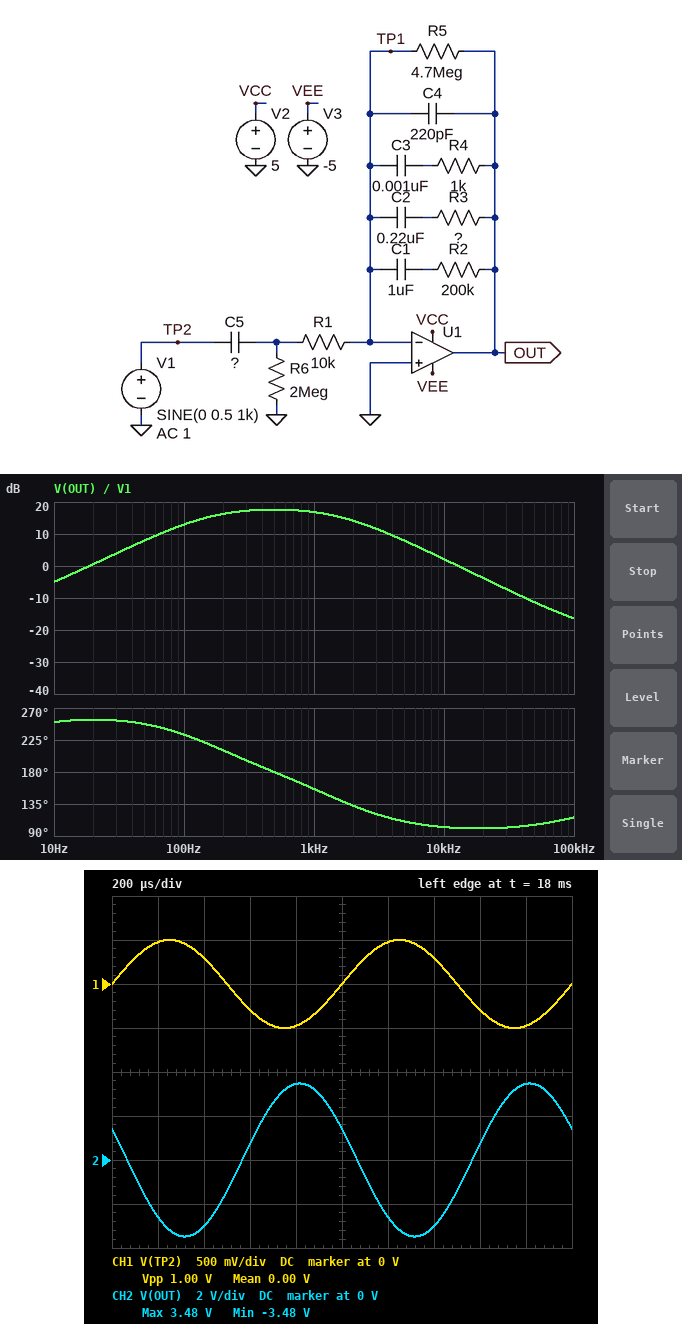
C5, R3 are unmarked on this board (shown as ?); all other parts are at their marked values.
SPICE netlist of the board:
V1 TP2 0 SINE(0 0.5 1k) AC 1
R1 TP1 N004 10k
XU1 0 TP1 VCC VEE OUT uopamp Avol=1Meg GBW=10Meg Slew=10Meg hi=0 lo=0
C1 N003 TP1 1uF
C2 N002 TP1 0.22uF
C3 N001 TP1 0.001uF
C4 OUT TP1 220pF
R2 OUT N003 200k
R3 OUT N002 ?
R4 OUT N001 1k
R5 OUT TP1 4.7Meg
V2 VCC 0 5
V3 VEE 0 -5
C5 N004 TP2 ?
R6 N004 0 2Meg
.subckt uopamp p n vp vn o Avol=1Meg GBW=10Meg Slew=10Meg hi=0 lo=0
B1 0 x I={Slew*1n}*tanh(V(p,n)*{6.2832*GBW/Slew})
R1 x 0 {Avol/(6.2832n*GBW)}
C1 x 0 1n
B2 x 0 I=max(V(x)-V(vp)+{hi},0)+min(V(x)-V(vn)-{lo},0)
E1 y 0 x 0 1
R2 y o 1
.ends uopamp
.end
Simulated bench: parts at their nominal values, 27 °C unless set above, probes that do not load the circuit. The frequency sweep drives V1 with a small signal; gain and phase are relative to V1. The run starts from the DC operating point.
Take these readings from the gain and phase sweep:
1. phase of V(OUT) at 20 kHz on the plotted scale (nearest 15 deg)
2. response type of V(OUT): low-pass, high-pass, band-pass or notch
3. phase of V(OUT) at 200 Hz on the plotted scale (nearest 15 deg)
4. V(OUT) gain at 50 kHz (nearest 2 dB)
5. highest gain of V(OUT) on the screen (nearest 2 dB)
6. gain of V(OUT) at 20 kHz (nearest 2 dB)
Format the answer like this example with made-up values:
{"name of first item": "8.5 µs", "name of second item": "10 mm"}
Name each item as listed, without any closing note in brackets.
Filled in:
{"phase of V(OUT) at 20 kHz on the plotted scale": "105 deg", "response type of V(OUT): low-pass, high-pass, band-pass or notch": "band-pass", "phase of V(OUT) at 200 Hz on the plotted scale": "210 deg", "V(OUT) gain at 50 kHz": "-12 dB", "highest gain of V(OUT) on the screen": "18 dB", "gain of V(OUT) at 20 kHz": "-4 dB"}
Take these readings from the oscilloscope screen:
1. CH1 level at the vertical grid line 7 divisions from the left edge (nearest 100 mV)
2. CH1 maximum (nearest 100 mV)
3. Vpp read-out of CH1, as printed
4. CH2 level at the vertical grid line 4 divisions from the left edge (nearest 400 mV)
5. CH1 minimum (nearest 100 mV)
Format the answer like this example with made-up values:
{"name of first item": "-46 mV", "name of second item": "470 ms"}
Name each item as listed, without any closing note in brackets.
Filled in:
{"CH1 level at the vertical grid line 7 divisions from the left edge": "300 mV", "CH1 maximum": "500 mV", "Vpp read-out of CH1, as printed": "1.00 V", "CH2 level at the vertical grid line 4 divisions from the left edge": "3.6 V", "CH1 minimum": "-500 mV"}
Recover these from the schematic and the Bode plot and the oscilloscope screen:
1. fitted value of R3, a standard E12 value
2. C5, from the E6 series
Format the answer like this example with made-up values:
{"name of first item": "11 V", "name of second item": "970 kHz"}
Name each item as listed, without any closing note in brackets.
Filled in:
{"fitted value of R3, a standard E12 value": "150 kΩ", "C5, from the E6 series": "100 nF"}
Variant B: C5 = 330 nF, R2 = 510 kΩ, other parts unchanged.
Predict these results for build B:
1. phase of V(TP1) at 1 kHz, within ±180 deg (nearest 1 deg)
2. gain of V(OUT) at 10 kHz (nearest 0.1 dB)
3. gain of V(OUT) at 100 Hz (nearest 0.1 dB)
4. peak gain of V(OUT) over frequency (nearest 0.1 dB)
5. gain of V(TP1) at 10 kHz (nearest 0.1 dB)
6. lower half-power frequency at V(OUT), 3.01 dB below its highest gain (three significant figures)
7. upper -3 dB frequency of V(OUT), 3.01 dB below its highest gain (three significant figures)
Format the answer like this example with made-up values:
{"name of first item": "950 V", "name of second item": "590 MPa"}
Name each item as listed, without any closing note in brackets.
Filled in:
{"phase of V(TP1) at 1 kHz, within ±180 deg": "51 deg", "gain of V(OUT) at 10 kHz": "2.2 dB", "gain of V(OUT) at 100 Hz": "20.1 dB", "peak gain of V(OUT) over frequency": "20.7 dB", "gain of V(TP1) at 10 kHz": "-57.8 dB", "lower half-power frequency at V(OUT), 3.01 dB below its highest gain": "44.4 Hz", "upper -3 dB frequency of V(OUT), 3.01 dB below its highest gain": "1.24 kHz"}
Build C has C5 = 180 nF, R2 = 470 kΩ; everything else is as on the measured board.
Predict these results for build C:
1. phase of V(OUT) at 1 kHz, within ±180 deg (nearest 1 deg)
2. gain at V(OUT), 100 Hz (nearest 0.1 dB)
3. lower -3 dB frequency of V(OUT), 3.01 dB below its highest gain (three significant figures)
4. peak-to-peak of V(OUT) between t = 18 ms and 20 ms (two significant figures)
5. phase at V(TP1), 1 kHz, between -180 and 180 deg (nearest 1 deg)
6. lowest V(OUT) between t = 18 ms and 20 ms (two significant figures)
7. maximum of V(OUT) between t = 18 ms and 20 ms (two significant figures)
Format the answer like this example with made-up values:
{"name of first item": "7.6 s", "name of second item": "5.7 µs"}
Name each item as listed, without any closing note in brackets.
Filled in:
{"phase of V(OUT) at 1 kHz, within ±180 deg": "145 deg", "gain at V(OUT), 100 Hz": "18.3 dB", "lower -3 dB frequency of V(OUT), 3.01 dB below its highest gain": "77.6 Hz", "peak-to-peak of V(OUT) between t = 18 ms and 20 ms": "8.4 V", "phase at V(TP1), 1 kHz, between -180 and 180 deg": "54 deg", "lowest V(OUT) between t = 18 ms and 20 ms": "-4.2 V", "maximum of V(OUT) between t = 18 ms and 20 ms": "4.2 V"}
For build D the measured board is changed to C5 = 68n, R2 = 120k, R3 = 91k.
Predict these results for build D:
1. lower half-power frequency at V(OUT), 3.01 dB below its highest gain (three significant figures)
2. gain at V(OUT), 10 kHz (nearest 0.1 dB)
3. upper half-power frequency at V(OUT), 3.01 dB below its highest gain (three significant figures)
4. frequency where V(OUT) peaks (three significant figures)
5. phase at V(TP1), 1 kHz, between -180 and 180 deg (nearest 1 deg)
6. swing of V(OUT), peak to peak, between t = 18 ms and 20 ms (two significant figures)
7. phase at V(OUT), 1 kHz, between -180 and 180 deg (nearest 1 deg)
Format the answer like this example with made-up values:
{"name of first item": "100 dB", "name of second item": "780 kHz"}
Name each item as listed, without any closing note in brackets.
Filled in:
{"lower half-power frequency at V(OUT), 3.01 dB below its highest gain": "200 Hz", "gain at V(OUT), 10 kHz": "1.9 dB", "upper half-power frequency at V(OUT), 3.01 dB below its highest gain": "2.95 kHz", "frequency where V(OUT) peaks": "769 Hz", "phase at V(TP1), 1 kHz, between -180 and 180 deg": "81 deg", "swing of V(OUT), peak to peak, between t = 18 ms and 20 ms": "4.6 V", "phase at V(OUT), 1 kHz, between -180 and 180 deg": "172 deg"}
